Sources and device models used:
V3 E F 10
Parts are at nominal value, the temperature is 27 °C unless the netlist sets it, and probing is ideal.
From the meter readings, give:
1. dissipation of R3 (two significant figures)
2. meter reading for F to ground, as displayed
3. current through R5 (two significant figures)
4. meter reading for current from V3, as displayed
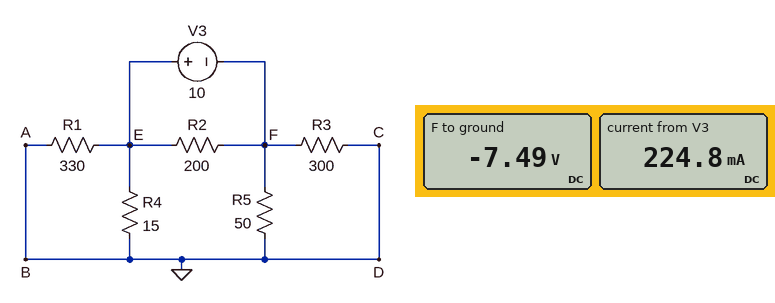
190 mW
-7.49 V
150 mA
224.8 mA
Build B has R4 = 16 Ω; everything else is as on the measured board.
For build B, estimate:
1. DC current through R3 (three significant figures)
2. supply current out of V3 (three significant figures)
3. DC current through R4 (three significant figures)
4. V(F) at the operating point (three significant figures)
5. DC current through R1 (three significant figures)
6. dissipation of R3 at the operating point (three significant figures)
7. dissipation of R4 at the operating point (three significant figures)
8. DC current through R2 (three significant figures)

24.6 mA
222 mA
164 mA
-7.37 V
7.96 mA
181 mW
431 mW
50.0 mA
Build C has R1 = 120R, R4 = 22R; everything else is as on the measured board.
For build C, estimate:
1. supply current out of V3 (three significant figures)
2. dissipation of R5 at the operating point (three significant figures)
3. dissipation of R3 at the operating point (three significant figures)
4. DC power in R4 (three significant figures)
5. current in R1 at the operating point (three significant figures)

213 mA
973 mW
162 mW
416 mW
25.2 mA
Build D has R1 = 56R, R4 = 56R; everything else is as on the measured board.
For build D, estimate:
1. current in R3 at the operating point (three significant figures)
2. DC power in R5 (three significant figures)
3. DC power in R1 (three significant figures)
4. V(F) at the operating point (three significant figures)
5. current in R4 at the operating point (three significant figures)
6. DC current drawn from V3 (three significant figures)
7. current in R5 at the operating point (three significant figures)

20.2 mA
732 mW
279 mW
-6.05 V
70.6 mA
191 mA
121 mA
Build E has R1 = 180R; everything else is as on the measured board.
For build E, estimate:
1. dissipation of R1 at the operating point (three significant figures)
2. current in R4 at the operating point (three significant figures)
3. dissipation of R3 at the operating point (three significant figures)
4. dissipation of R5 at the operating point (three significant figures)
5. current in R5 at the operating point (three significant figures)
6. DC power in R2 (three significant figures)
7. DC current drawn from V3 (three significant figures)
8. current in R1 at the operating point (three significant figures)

33.1 mW
163 mA
190 mW
1.14 W
151 mA
500 mW
226 mA
13.6 mA
